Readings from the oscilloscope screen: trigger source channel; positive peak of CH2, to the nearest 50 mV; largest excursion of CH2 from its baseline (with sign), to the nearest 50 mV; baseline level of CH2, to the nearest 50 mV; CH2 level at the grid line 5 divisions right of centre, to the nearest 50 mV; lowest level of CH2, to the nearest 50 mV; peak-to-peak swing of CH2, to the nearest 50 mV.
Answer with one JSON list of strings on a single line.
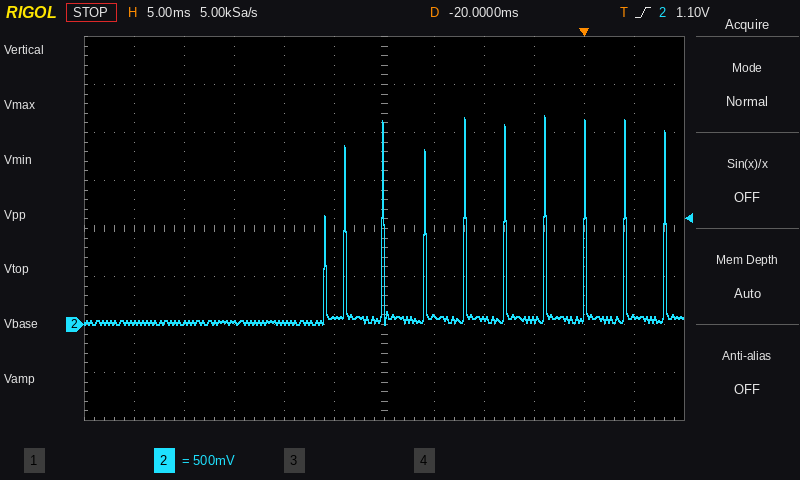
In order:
["CH2", "2.20 V", "+2.15 V", "50 mV", "100 mV", "0 mV", "2.20 V"]
